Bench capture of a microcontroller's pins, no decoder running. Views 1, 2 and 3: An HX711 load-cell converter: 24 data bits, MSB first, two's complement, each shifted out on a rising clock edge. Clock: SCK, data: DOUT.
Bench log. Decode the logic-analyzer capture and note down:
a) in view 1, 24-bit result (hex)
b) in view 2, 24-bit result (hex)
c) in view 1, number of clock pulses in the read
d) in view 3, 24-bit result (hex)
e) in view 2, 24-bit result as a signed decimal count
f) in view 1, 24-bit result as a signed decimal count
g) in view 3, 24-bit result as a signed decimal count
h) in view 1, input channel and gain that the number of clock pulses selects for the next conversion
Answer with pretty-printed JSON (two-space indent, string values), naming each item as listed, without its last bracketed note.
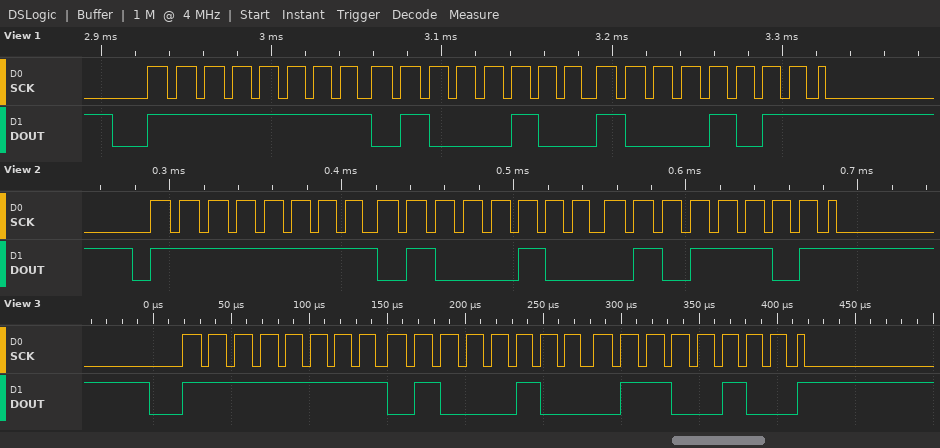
{
  "in view 1, 24-bit result": "0xFF448B",
  "in view 2, 24-bit result": "0xFF445D",
  "in view 1, number of clock pulses in the read": "25",
  "in view 3, 24-bit result": "0xFF4464",
  "in view 2, 24-bit result as a signed decimal count": "-48035",
  "in view 1, 24-bit result as a signed decimal count": "-47989",
  "in view 3, 24-bit result as a signed decimal count": "-48028",
  "in view 1, input channel and gain that the number of clock pulses selects for the next conversion": "channel A, gain 128"
}
